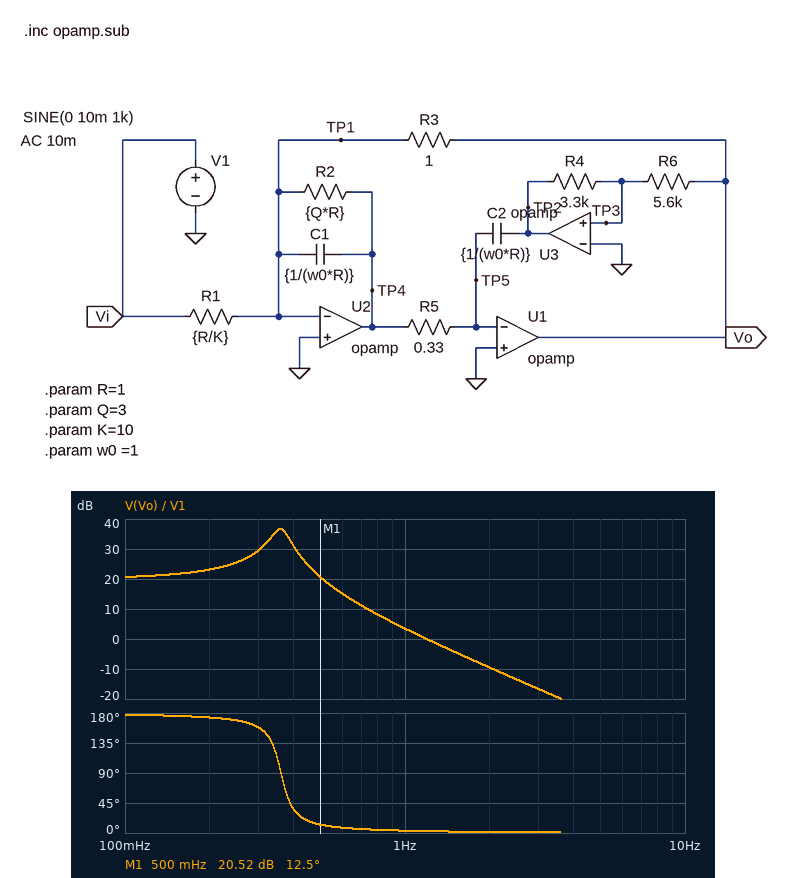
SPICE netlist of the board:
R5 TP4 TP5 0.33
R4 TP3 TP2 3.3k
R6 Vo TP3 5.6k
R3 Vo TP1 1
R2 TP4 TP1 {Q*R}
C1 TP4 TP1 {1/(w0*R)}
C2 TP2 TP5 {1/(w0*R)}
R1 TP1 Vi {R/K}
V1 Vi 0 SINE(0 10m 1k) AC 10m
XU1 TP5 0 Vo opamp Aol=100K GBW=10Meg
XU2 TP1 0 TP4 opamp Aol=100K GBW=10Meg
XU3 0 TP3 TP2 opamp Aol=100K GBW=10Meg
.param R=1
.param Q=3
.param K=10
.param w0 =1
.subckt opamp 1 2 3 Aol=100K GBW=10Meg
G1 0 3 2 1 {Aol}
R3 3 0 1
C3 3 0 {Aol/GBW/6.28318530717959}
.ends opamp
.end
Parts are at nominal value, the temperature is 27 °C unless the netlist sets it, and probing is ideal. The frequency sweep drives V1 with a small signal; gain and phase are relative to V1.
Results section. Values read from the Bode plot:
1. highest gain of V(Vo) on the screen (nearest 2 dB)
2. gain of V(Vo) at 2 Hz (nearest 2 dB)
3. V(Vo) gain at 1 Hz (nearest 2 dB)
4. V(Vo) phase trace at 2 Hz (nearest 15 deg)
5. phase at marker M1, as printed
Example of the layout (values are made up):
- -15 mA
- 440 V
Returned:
- 36 dB
- -10 dB
- 4 dB
- 0 deg
- 12.5 deg
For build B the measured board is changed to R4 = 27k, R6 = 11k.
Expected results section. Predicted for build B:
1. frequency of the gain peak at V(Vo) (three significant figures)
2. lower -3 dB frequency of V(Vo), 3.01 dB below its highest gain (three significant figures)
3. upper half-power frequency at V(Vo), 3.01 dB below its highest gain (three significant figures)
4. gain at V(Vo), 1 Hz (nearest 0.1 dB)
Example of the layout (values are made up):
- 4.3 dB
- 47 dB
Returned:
- 173 mHz
- 143 mHz
- 198 mHz
- -9.8 dB
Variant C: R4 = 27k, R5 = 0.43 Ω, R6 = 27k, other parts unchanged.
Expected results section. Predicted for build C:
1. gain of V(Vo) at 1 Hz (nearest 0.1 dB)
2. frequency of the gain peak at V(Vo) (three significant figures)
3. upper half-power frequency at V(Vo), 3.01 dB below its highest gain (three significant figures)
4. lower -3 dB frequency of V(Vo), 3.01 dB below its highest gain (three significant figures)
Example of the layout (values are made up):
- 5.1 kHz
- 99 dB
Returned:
- -4.1 dB
- 240 mHz
- 265 mHz
- 211 mHz
